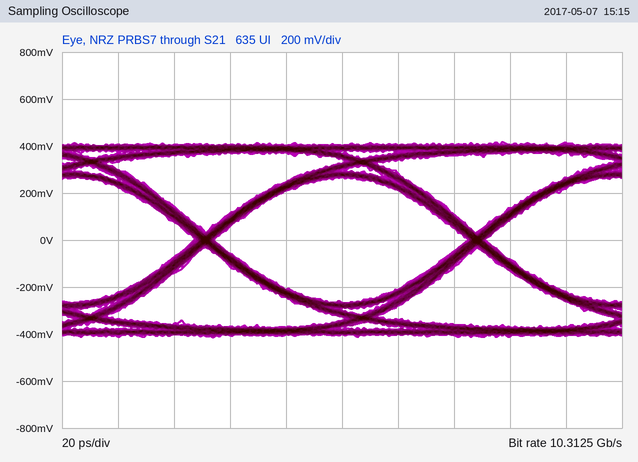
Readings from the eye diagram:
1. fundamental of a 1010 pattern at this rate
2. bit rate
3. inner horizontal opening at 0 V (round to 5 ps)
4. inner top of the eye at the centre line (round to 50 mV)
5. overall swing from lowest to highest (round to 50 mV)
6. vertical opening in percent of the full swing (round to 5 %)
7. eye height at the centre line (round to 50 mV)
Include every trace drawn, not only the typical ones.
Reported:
5.15625 GHz
10.3125 Gb/s
90 ps
250 mV
850 mV
65 %
550 mV
